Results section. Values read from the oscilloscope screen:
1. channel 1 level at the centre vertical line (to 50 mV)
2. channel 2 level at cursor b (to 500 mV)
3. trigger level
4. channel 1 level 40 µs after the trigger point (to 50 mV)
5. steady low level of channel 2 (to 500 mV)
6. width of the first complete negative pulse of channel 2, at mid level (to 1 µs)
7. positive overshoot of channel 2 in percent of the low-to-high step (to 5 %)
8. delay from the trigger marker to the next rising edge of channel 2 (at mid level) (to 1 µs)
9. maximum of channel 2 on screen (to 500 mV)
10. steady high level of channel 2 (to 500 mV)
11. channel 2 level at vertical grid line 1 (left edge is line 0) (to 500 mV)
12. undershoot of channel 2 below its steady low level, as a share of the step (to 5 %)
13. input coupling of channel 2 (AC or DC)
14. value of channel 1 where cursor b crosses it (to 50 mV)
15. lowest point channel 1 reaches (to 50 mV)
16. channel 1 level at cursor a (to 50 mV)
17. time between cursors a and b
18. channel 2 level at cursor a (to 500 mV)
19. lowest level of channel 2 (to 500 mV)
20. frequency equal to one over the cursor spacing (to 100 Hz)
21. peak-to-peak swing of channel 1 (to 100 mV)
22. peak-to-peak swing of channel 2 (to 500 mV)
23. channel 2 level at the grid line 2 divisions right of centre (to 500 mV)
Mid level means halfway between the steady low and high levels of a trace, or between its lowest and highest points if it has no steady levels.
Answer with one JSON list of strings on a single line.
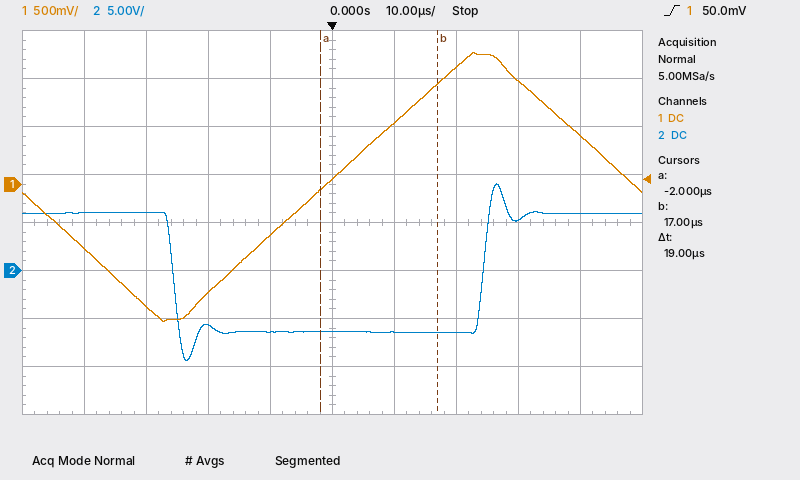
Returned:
["50 mV", "-6.5 V", "50.0 mV", "500 mV", "-6.5 V", "50 µs", "25 %", "24 µs", "9.0 V", "6.0 V", "6.0 V", "25 %", "DC", "1.05 V", "-1.45 V", "-50 mV", "19 µs", "-6.5 V", "-9.5 V", "52.6 kHz", "2.80 V", "18.5 V", "-6.5 V"]
